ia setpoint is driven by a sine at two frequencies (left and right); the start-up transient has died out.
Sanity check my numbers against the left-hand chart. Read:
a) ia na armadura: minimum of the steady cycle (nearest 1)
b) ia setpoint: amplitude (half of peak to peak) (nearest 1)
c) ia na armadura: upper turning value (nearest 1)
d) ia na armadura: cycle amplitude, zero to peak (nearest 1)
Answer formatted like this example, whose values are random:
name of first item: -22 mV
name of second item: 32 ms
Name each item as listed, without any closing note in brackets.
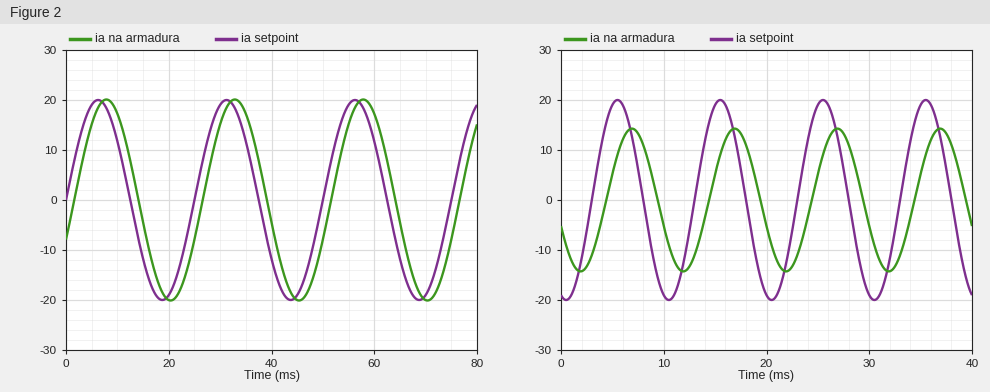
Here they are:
ia na armadura: minimum of the steady cycle: -20
ia setpoint: amplitude (half of peak to peak): 20
ia na armadura: upper turning value: 20
ia na armadura: cycle amplitude, zero to peak: 20
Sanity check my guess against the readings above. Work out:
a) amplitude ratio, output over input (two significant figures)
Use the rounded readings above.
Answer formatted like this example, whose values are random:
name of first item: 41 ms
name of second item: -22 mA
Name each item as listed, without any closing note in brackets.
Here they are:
amplitude ratio, output over input: 1.0
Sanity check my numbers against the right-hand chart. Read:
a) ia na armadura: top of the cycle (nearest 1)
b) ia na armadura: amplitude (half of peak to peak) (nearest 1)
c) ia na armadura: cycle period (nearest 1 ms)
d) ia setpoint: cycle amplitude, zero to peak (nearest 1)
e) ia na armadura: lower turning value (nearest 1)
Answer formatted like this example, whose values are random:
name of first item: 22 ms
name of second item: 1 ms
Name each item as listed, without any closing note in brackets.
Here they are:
ia na armadura: top of the cycle: 14
ia na armadura: amplitude (half of peak to peak): 14
ia na armadura: cycle period: 10 ms
ia setpoint: cycle amplitude, zero to peak: 20
ia na armadura: lower turning value: -14
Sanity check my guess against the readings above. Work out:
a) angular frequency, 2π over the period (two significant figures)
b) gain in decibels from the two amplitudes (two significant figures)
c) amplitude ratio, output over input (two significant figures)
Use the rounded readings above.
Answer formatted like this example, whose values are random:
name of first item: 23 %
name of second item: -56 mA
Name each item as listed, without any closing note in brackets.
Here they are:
angular frequency, 2π over the period: 0.63 rad/ms
gain in decibels from the two amplitudes: -3.1 dB
amplitude ratio, output over input: 0.70
